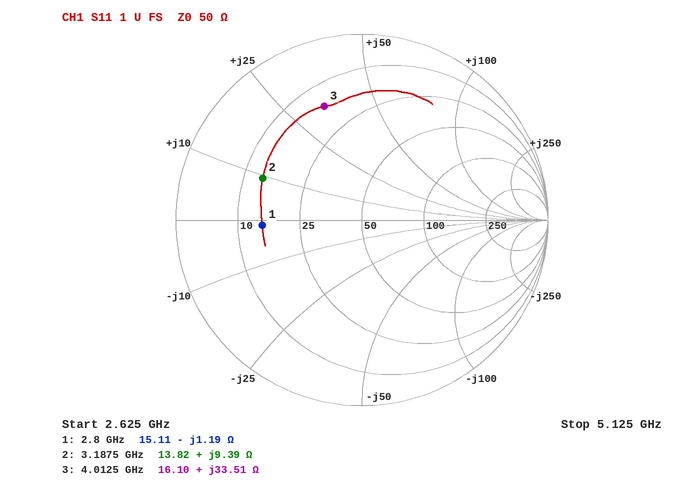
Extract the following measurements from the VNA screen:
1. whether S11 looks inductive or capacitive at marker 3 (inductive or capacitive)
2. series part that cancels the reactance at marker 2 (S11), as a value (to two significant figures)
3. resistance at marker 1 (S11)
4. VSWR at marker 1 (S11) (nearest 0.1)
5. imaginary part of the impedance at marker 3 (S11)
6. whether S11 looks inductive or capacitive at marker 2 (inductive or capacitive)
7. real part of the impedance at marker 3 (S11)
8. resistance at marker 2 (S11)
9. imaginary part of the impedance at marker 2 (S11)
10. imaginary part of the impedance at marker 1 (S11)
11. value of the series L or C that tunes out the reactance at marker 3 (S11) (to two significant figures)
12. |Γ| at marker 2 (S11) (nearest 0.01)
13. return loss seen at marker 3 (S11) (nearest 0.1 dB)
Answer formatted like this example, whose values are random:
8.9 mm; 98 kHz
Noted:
inductive; 5.3 pF; 15.11 Ω; 3.3; +33.51 Ω; inductive; 16.10 Ω; 13.82 Ω; +9.39 Ω; -1.19 Ω; 1.2 pF; 0.58; 3.8 dB
